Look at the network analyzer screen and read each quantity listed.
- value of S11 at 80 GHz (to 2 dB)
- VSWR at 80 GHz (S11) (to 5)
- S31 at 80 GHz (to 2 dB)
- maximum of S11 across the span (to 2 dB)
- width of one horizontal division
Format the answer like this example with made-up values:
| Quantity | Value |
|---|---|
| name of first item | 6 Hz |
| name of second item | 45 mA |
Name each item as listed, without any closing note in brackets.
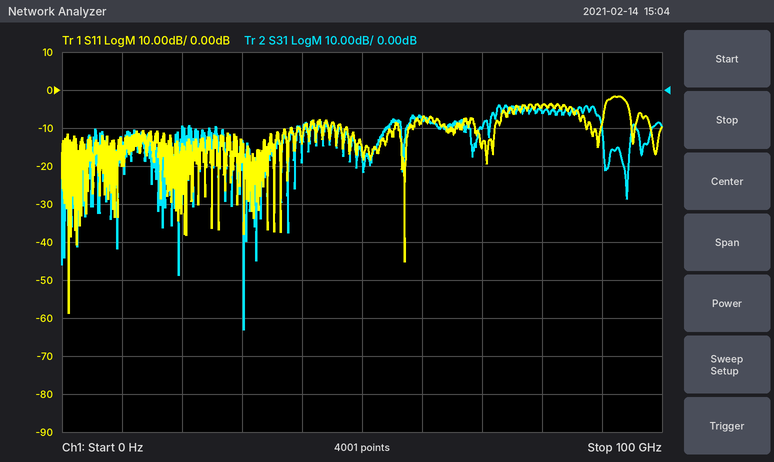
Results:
| Quantity | Value |
|---|---|
| value of S11 at 80 GHz | -4 dB |
| VSWR at 80 GHz (S11) | 5 |
| S31 at 80 GHz | -6 dB |
| maximum of S11 across the span | -2 dB |
| width of one horizontal division | 10 GHz |
